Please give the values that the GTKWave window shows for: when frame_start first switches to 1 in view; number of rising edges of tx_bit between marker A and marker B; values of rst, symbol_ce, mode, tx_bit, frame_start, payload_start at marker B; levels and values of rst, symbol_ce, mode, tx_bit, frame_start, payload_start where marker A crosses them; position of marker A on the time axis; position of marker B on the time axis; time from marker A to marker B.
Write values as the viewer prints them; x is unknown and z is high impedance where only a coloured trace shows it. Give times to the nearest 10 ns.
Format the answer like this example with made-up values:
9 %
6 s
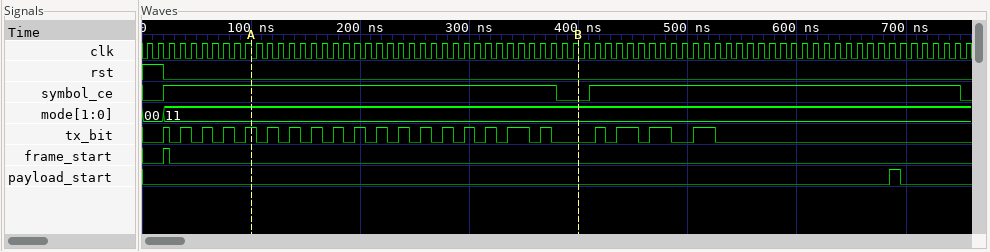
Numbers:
20 ns
13
rst=0, symbol_ce=0, mode=11, tx_bit=0, frame_start=0, payload_start=0
rst=0, symbol_ce=1, mode=11, tx_bit=1, frame_start=0, payload_start=0
100 ns
400 ns
300 ns
